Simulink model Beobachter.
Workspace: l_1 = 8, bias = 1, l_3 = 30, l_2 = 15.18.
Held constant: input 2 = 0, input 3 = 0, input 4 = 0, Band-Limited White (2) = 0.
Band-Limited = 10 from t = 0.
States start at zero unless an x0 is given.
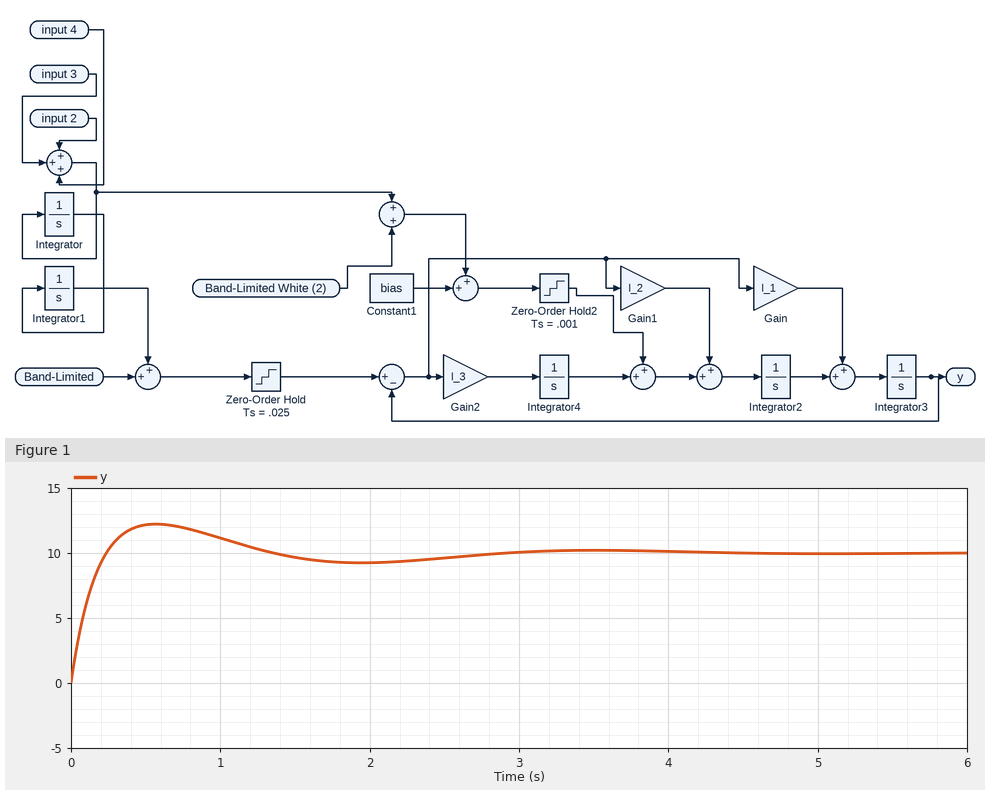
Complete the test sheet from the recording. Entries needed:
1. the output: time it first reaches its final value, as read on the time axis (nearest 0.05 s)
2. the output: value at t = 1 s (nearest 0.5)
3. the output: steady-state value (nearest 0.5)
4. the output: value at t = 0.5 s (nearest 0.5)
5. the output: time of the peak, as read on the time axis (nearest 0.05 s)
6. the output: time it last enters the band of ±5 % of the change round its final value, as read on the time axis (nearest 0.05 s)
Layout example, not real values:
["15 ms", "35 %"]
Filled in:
["0.25 s", "11.0", "10.0", "12.0", "0.55 s", "2.40 s"]
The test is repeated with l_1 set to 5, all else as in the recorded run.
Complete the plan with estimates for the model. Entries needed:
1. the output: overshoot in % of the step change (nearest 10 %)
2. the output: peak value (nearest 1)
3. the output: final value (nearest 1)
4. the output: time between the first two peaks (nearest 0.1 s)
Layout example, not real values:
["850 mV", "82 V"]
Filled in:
["40 %", "14", "10", "2.1 s"]
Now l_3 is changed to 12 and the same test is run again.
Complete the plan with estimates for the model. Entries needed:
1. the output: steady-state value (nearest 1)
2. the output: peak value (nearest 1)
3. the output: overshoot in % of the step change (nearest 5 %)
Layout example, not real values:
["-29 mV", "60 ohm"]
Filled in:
["10", "12", "15 %"]
